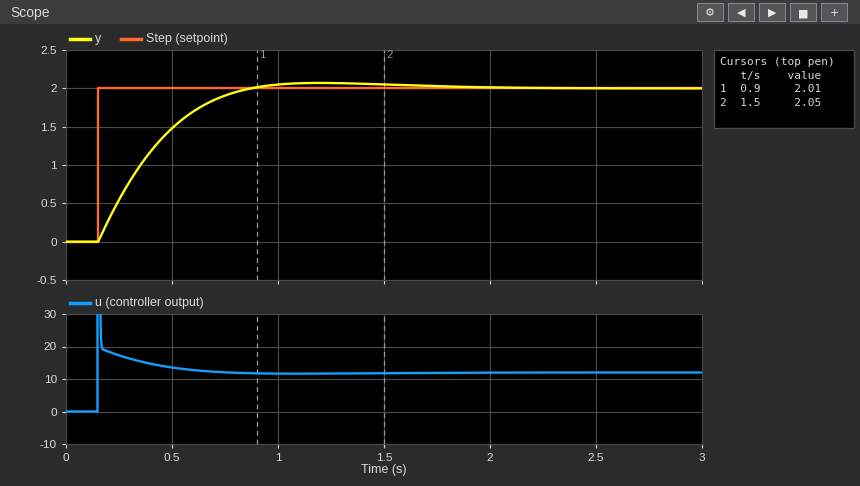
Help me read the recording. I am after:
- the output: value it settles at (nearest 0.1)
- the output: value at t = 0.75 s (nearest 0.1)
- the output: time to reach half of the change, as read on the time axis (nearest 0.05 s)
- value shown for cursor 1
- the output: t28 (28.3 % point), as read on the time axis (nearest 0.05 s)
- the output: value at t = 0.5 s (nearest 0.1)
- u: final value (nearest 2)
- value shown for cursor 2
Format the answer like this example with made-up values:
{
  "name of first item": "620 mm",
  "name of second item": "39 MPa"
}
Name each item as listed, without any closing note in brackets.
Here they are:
{
  "the output: value it settles at": "2.0",
  "the output: value at t = 0.75 s": "1.9",
  "the output: time to reach half of the change, as read on the time axis": "0.35 s",
  "value shown for cursor 1": "2.01",
  "the output: t28 (28.3 % point), as read on the time axis": "0.25 s",
  "the output: value at t = 0.5 s": "1.5",
  "u: final value": "12",
  "value shown for cursor 2": "2.05"
}
